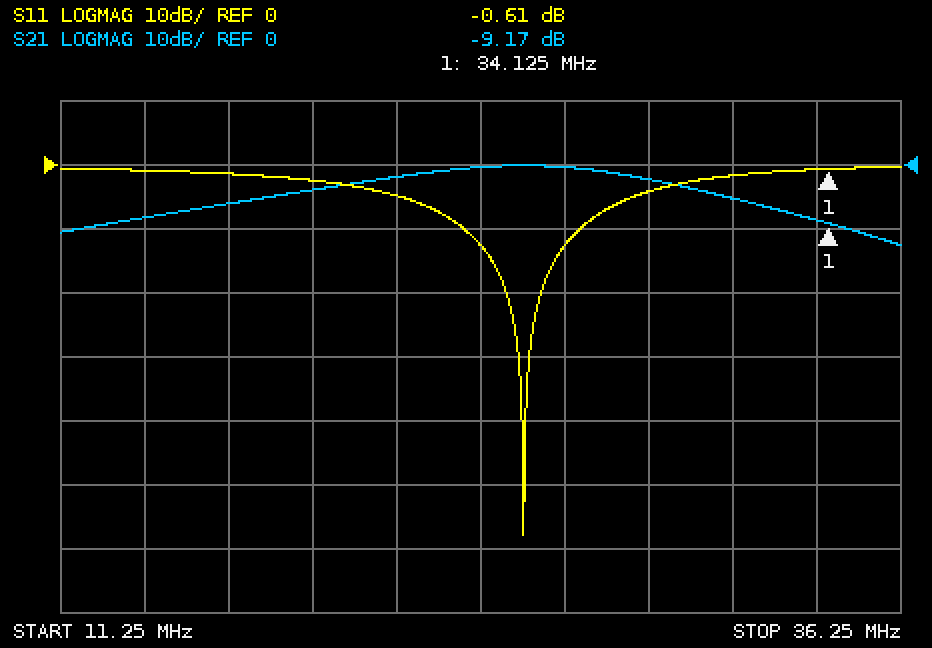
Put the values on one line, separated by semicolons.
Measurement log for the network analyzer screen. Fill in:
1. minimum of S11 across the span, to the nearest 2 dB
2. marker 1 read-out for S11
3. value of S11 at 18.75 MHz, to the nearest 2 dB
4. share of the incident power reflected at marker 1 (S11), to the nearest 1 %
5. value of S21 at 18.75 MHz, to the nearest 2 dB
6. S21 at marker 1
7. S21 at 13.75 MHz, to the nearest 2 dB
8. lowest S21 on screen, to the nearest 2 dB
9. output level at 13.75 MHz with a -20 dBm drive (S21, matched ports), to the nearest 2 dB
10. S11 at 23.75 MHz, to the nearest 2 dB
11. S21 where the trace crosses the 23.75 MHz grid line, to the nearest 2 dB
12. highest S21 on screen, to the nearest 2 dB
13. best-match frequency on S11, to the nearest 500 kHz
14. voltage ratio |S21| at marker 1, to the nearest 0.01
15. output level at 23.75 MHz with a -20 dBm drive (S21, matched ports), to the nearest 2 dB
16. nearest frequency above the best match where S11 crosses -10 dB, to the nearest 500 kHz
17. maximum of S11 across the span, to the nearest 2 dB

-58 dB; -0.61 dB; -2 dB; 87 %; -4 dB; -9.17 dB; -8 dB; -12 dB; -28 dBm; -12 dB; 0 dB; 0 dB; 25.0 MHz; 0.35; -20 dBm; 26.5 MHz; 0 dB
